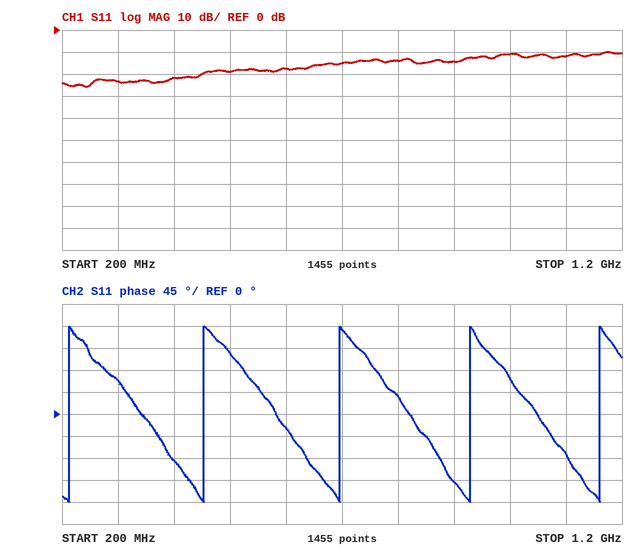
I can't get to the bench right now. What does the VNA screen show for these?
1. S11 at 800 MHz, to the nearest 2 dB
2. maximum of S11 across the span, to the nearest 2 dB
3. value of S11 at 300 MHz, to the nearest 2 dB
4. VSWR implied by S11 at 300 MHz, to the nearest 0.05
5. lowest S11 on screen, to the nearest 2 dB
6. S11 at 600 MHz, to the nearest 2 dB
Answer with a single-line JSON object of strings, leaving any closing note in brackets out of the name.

{"S11 at 800 MHz, to the nearest 2 dB": "-14 dB", "maximum of S11 across the span, to the nearest 2 dB": "-10 dB", "value of S11 at 300 MHz, to the nearest 2 dB": "-24 dB", "VSWR implied by S11 at 300 MHz, to the nearest 0.05": "1.15", "lowest S11 on screen, to the nearest 2 dB": "-26 dB", "S11 at 600 MHz, to the nearest 2 dB": "-18 dB"}
